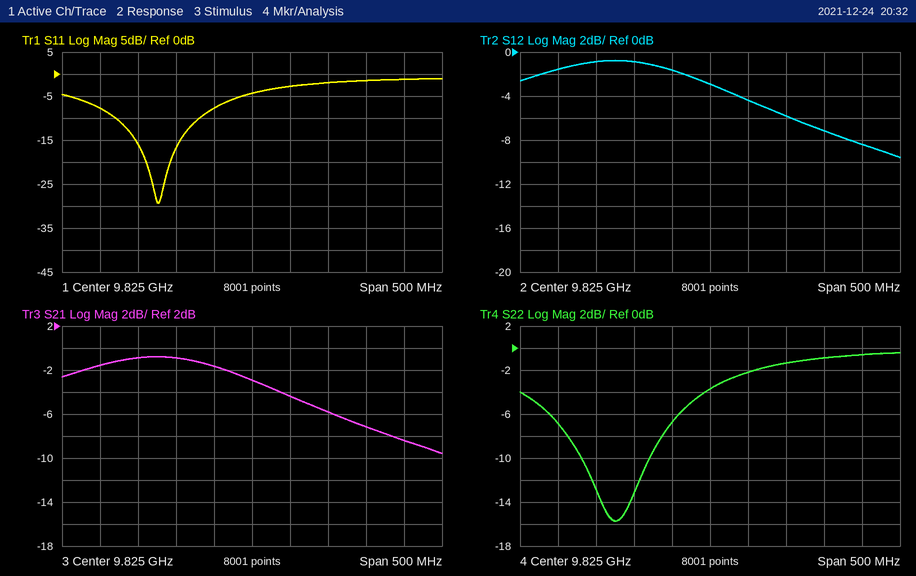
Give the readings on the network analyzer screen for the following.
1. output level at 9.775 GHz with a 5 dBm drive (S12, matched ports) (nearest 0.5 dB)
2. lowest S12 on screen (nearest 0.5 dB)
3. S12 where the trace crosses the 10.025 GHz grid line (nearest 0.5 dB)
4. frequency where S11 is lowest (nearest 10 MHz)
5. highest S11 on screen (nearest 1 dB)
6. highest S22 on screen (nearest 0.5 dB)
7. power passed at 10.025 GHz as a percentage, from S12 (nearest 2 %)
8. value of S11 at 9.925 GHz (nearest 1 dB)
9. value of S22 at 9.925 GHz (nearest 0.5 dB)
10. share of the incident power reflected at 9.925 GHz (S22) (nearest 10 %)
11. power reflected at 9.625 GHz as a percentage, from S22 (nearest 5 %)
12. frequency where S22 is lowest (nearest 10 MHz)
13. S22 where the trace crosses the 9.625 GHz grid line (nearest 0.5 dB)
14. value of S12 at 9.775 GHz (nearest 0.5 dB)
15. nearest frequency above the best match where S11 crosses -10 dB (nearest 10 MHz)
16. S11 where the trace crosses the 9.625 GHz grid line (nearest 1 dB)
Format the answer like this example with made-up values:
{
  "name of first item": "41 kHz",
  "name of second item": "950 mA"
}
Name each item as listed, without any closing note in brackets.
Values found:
{
  "output level at 9.775 GHz with a 5 dBm drive (S12, matched ports)": "3.5 dBm",
  "lowest S12 on screen": "-9.5 dB",
  "S12 where the trace crosses the 10.025 GHz grid line": "-8.5 dB",
  "frequency where S11 is lowest": "9.70 GHz",
  "highest S11 on screen": "-1 dB",
  "highest S22 on screen": "-0.5 dB",
  "power passed at 10.025 GHz as a percentage, from S12": "14 %",
  "value of S11 at 9.925 GHz": "-2 dB",
  "value of S22 at 9.925 GHz": "-1.5 dB",
  "share of the incident power reflected at 9.925 GHz (S22)": "70 %",
  "power reflected at 9.625 GHz as a percentage, from S22": "20 %",
  "frequency where S22 is lowest": "9.70 GHz",
  "S22 where the trace crosses the 9.625 GHz grid line": "-7.0 dB",
  "value of S12 at 9.775 GHz": "-1.5 dB",
  "nearest frequency above the best match where S11 crosses -10 dB": "9.76 GHz",
  "S11 where the trace crosses the 9.625 GHz grid line": "-8 dB"
}
